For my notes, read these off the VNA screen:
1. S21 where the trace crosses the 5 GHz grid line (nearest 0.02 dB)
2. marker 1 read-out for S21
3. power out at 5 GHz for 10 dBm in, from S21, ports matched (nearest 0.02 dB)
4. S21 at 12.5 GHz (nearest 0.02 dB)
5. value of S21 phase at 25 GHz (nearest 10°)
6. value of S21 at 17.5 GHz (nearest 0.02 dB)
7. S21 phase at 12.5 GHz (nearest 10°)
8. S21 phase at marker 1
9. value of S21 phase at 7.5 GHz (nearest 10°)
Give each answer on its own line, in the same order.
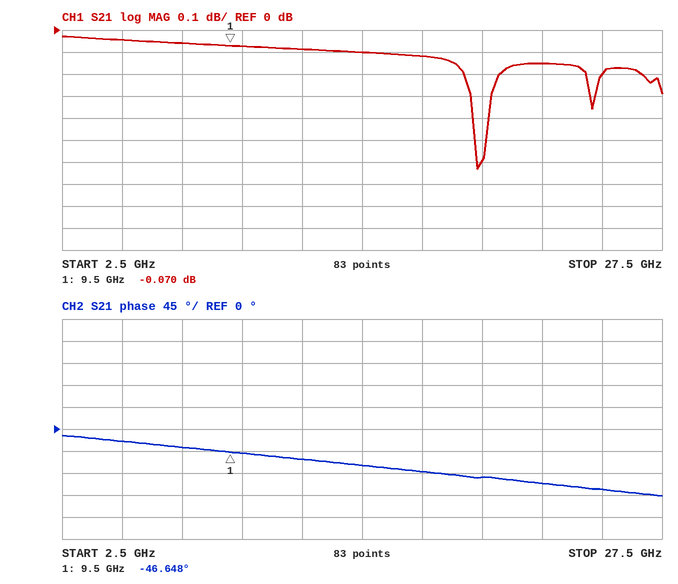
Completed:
-0.04 dB
-0.070 dB
9.96 dBm
-0.08 dB
-120°
-0.12 dB
-60°
-46.648°
-40°
